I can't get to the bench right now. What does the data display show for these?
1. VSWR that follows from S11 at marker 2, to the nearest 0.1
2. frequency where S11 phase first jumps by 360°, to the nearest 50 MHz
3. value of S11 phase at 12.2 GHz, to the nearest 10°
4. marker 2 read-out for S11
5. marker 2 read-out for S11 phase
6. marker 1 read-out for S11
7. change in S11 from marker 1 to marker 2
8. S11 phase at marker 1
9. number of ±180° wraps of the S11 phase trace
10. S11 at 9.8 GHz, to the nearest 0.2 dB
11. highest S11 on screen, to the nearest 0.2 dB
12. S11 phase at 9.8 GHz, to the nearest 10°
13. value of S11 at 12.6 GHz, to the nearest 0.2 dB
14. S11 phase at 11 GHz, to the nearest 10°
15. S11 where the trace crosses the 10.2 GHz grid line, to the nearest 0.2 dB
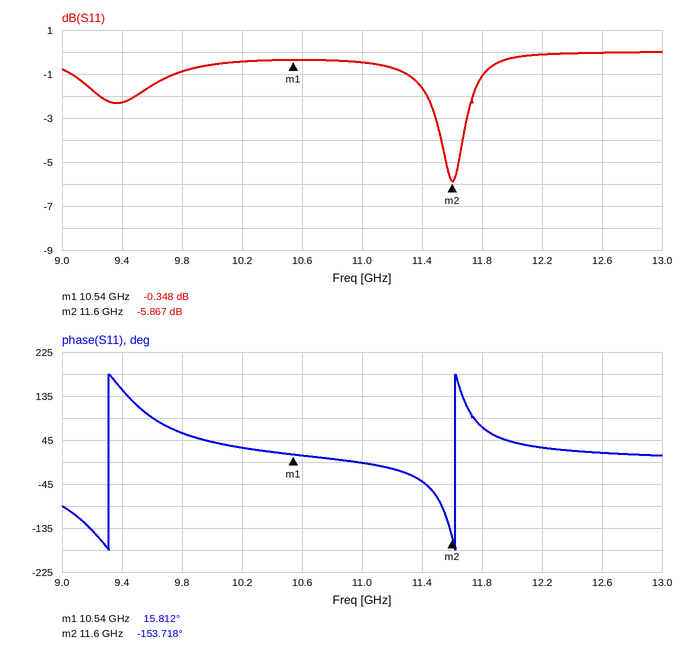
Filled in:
3.1
9.30 GHz
30°
-5.867 dB
-153.718°
-0.348 dB
-5.519 dB
15.812°
2
-0.8 dB
0.0 dB
60°
0.0 dB
0°
-0.4 dB
